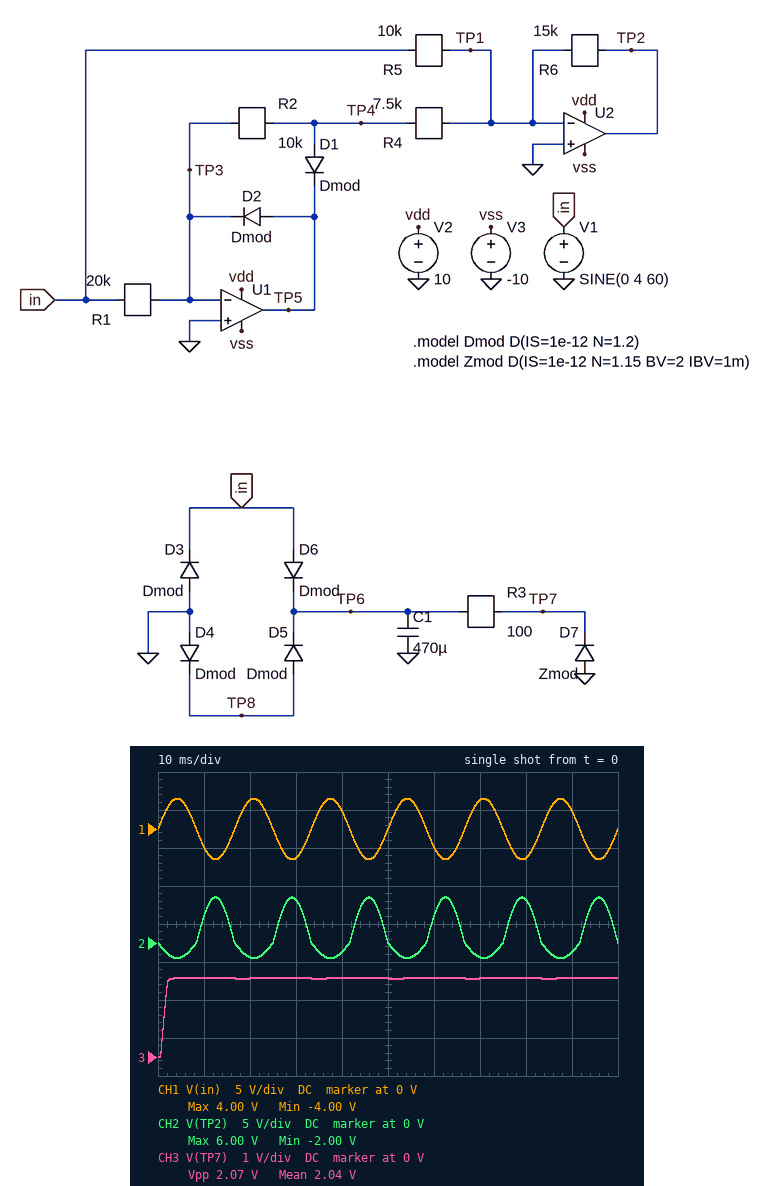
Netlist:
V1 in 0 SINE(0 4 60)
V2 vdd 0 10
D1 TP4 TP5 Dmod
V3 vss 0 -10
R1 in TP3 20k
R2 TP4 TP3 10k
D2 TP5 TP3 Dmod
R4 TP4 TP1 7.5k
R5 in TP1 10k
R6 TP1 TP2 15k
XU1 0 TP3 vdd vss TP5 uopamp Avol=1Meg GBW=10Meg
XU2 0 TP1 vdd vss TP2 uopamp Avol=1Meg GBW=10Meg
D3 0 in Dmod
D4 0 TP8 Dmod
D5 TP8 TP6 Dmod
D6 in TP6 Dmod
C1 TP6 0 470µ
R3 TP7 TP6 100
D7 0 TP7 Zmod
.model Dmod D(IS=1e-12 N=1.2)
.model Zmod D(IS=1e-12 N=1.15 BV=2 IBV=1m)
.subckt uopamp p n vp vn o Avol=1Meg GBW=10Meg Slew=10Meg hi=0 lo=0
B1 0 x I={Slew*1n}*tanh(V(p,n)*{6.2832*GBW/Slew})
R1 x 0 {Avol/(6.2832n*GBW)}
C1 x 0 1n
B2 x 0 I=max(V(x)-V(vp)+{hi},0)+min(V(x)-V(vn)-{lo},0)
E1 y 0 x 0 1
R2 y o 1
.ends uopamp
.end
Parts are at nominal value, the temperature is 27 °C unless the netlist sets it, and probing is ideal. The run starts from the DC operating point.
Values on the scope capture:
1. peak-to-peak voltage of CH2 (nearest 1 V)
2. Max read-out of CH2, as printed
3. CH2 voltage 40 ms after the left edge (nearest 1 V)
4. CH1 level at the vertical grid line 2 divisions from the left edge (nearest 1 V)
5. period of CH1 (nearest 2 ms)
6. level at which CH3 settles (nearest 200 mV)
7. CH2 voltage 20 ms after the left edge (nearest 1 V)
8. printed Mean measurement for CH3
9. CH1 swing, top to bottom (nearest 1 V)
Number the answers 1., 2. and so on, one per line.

1. 8 V
2. 6.00 V
3. -1 V
4. 4 V
5. 16 ms
6. 2.0 V
7. -2 V
8. 2.04 V
9. 8 V
